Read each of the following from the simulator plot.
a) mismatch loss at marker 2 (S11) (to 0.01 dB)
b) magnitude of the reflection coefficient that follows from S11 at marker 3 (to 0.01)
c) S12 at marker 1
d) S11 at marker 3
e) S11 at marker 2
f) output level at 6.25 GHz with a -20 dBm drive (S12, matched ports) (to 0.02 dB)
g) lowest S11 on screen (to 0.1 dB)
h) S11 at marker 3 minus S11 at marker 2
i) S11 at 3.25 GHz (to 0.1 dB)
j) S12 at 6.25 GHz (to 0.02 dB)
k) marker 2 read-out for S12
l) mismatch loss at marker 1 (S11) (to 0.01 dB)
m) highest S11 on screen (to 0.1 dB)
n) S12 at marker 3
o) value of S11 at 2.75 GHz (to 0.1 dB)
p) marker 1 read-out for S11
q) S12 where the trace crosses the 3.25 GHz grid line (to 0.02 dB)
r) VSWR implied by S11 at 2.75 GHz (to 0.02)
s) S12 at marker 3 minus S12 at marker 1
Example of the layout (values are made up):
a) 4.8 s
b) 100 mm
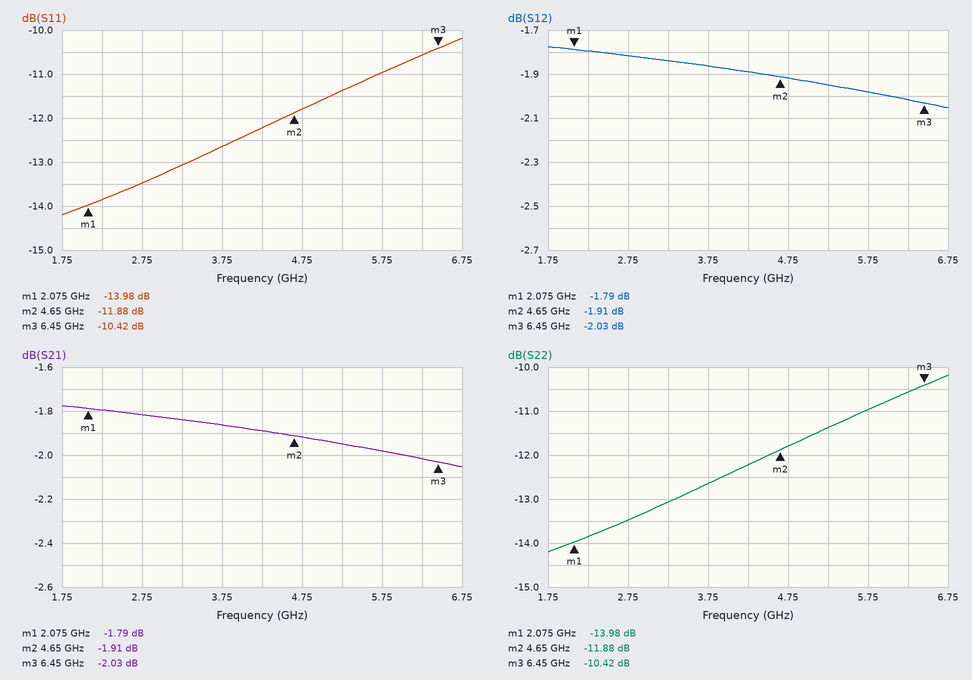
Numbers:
a) 0.29 dB
b) 0.30
c) -1.79 dB
d) -10.42 dB
e) -11.88 dB
f) -22.02 dBm
g) -14.2 dB
h) 1.46 dB
i) -13.1 dB
j) -2.02 dB
k) -1.91 dB
l) 0.18 dB
m) -10.2 dB
n) -2.03 dB
o) -13.5 dB
p) -13.98 dB
q) -1.84 dB
r) 1.54
s) -0.24 dB
